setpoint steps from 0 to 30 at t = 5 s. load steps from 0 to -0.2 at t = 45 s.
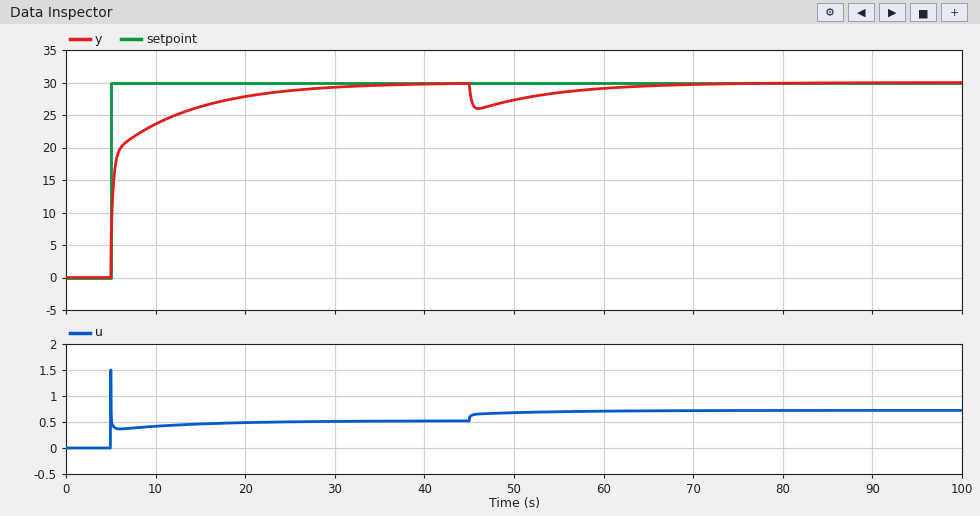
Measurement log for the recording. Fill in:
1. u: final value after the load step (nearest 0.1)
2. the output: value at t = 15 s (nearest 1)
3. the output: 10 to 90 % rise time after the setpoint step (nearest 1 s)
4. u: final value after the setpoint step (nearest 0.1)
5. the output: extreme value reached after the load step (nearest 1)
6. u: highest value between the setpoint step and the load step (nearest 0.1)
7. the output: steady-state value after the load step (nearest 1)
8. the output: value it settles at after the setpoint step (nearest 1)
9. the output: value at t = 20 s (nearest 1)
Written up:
0.7
26
12 s
0.5
26
1.5
30
30
28
